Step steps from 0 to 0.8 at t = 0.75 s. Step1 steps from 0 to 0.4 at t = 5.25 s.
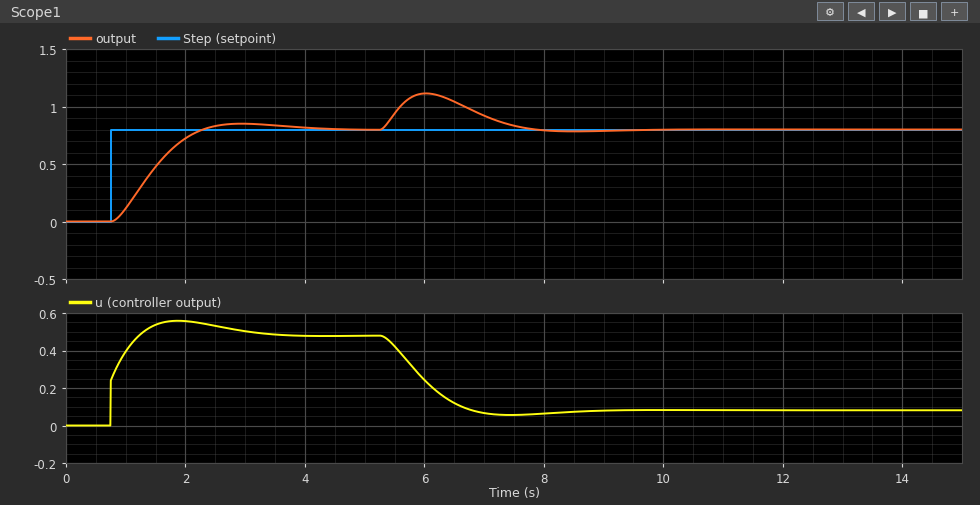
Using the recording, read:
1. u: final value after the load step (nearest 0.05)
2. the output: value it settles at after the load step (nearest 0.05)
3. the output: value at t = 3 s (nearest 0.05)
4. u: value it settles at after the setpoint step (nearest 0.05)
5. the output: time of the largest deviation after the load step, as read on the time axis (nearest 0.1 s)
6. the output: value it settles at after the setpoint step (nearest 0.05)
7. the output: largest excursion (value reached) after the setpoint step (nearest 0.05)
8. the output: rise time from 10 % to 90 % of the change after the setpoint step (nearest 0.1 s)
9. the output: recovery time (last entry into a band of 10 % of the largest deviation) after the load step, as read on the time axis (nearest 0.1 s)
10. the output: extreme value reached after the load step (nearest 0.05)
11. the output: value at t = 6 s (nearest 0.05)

0.10
0.80
0.85
0.50
6.0 s
0.80
0.85
1.0 s
7.5 s
1.10
1.10
